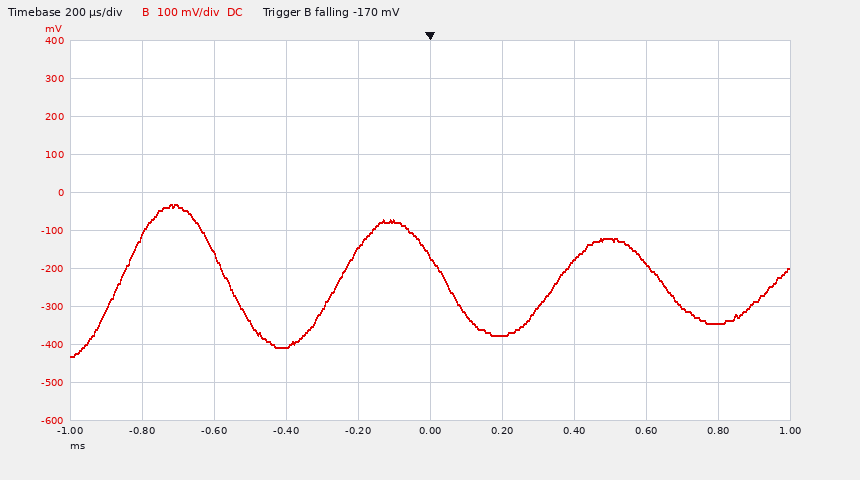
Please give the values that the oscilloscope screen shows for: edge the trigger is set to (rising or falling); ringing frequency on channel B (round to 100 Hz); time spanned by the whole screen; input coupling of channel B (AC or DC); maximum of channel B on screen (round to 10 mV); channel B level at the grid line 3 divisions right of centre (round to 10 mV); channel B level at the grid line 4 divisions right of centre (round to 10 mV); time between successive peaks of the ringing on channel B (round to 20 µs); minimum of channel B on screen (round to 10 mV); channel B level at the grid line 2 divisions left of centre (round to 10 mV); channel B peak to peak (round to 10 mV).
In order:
falling
1.7 kHz
2 ms
DC
-30 mV
-190 mV
-340 mV
600 µs
-430 mV
-410 mV
400 mV
